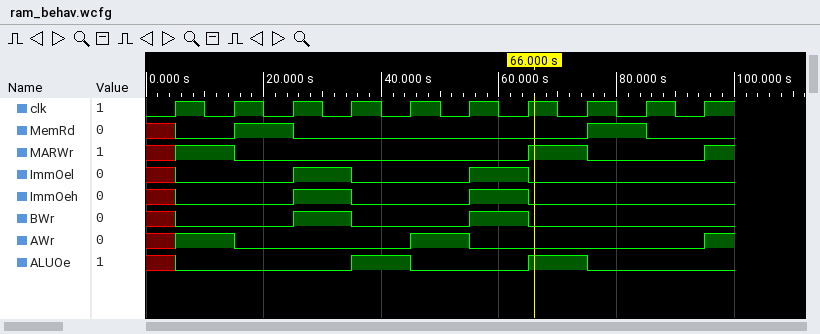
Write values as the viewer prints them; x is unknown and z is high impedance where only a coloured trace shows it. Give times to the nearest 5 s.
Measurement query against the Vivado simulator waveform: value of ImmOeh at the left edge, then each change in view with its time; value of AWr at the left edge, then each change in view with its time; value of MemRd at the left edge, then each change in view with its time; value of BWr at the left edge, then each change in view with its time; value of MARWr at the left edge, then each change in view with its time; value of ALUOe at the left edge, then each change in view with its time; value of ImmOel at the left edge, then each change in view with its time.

x, 0 at 5 s, 1 at 25 s, 0 at 35 s, 1 at 55 s, 0 at 65 s
x, 1 at 5 s, 0 at 15 s, 1 at 45 s, 0 at 55 s, 1 at 95 s
x, 0 at 5 s, 1 at 15 s, 0 at 25 s, 1 at 75 s, 0 at 85 s
x, 0 at 5 s, 1 at 25 s, 0 at 35 s, 1 at 55 s, 0 at 65 s
x, 1 at 5 s, 0 at 15 s, 1 at 65 s, 0 at 75 s, 1 at 95 s
x, 0 at 5 s, 1 at 35 s, 0 at 45 s, 1 at 65 s, 0 at 75 s
x, 0 at 5 s, 1 at 25 s, 0 at 35 s, 1 at 55 s, 0 at 65 s
